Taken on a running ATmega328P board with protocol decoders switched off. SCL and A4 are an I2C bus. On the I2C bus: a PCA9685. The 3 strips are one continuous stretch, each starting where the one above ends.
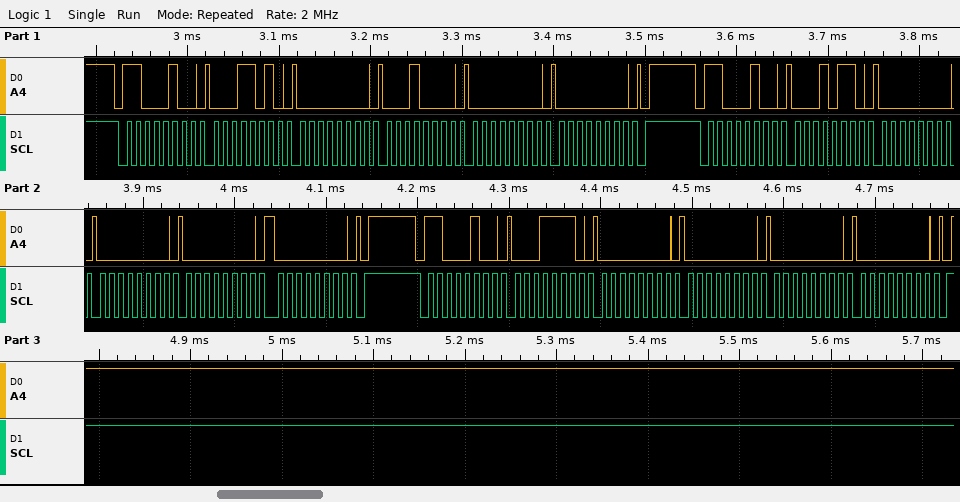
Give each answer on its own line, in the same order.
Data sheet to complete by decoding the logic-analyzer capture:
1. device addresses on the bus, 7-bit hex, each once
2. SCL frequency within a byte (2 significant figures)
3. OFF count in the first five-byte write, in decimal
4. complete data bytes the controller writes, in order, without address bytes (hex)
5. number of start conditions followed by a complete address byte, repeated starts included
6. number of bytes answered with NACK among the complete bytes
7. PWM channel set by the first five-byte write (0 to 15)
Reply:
0x62
100 kHz
0
1A 00 10 00 00 16 00 00 00 00 1E 00 00 00 00
3
0
5
